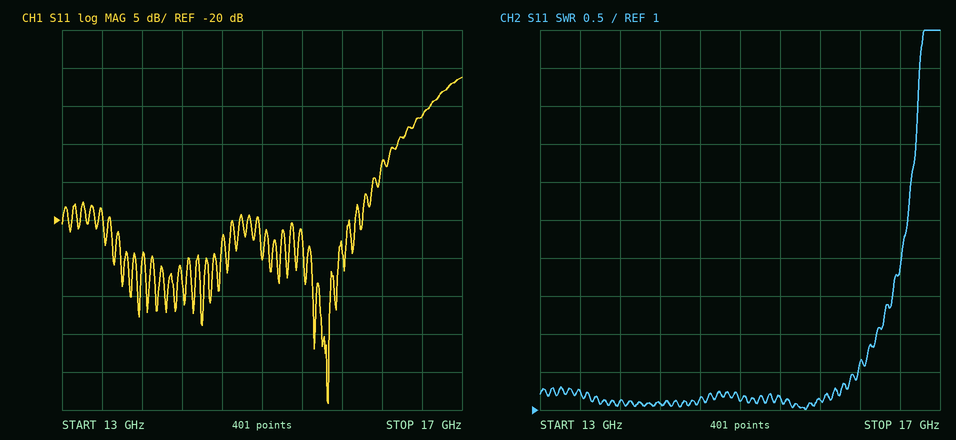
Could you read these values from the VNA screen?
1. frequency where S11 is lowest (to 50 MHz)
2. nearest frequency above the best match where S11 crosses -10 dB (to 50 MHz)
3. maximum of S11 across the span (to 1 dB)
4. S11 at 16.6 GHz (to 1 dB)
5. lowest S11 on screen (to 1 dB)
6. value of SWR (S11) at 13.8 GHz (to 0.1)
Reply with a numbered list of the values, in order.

1. 15.65 GHz
2. 16.35 GHz
3. -1 dB
4. -6 dB
5. -44 dB
6. 1.1
